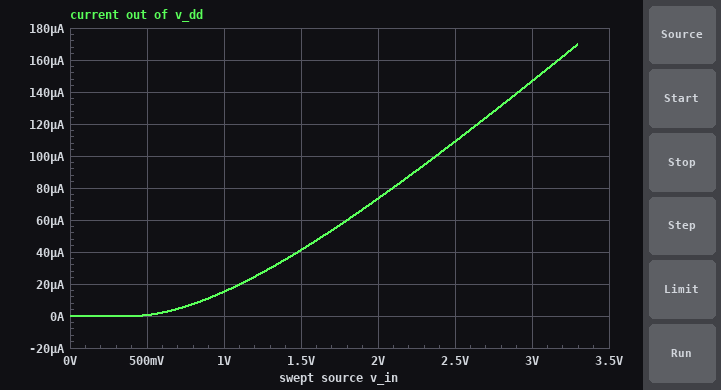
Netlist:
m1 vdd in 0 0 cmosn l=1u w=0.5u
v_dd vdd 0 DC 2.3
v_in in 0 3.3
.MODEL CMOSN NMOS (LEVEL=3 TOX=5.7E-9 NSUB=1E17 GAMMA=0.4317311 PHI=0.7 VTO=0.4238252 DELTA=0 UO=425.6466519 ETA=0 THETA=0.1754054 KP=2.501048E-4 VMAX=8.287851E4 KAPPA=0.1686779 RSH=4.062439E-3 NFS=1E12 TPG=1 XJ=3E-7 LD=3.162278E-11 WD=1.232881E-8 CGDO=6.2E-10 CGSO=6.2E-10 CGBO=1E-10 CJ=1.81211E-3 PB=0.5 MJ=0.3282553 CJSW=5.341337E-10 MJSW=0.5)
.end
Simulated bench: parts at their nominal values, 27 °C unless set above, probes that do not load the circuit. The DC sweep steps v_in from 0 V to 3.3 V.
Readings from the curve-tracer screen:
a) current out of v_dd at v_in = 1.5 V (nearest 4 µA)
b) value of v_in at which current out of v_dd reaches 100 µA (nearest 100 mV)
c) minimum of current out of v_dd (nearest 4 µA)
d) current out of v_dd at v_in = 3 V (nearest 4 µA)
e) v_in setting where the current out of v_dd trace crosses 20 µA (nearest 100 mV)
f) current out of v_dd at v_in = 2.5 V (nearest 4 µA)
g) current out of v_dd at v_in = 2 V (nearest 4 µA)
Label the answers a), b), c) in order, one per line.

a) 40 µA
b) 2.4 V
c) 0 A
d) 148 µA
e) 1.1 V
f) 108 µA
g) 72 µA
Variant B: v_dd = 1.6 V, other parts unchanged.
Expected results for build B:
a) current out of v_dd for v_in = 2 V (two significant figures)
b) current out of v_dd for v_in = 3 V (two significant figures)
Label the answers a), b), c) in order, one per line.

a) 72 µA
b) 140 µA
